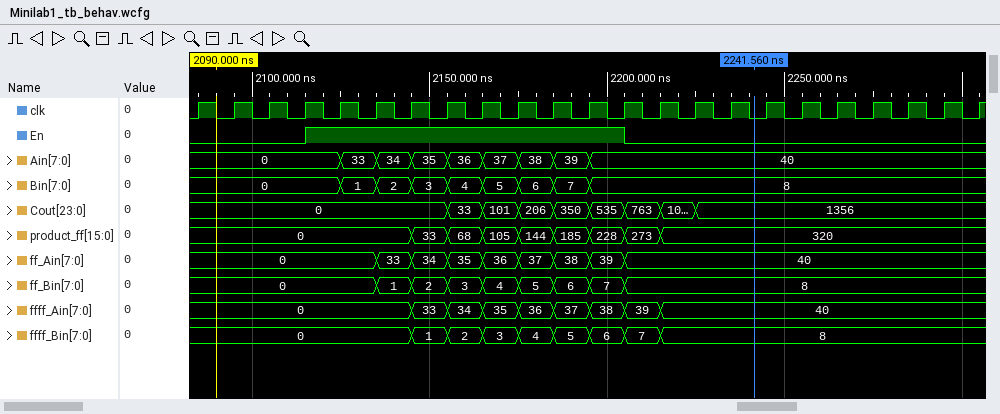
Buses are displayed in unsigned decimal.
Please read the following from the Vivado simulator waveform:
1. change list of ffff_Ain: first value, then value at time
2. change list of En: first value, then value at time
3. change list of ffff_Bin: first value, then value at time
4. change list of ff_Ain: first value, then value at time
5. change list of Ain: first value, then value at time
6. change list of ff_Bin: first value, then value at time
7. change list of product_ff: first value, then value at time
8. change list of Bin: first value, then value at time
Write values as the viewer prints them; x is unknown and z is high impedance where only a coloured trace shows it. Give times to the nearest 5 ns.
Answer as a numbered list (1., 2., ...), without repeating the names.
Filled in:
1. 0, 33 at 2145 ns, 34 at 2155 ns, 35 at 2165 ns, 36 at 2175 ns, 37 at 2185 ns, 38 at 2195 ns, 39 at 2205 ns, 40 at 2215 ns
2. 0, 1 at 2115 ns, 0 at 2205 ns
3. 0, 1 at 2145 ns, 2 at 2155 ns, 3 at 2165 ns, 4 at 2175 ns, 5 at 2185 ns, 6 at 2195 ns, 7 at 2205 ns, 8 at 2215 ns
4. 0, 33 at 2135 ns, 34 at 2145 ns, 35 at 2155 ns, 36 at 2165 ns, 37 at 2175 ns, 38 at 2185 ns, 39 at 2195 ns, 40 at 2205 ns
5. 0, 33 at 2125 ns, 34 at 2135 ns, 35 at 2145 ns, 36 at 2155 ns, 37 at 2165 ns, 38 at 2175 ns, 39 at 2185 ns, 40 at 2195 ns
6. 0, 1 at 2135 ns, 2 at 2145 ns, 3 at 2155 ns, 4 at 2165 ns, 5 at 2175 ns, 6 at 2185 ns, 7 at 2195 ns, 8 at 2205 ns
7. 0, 33 at 2145 ns, 68 at 2155 ns, 105 at 2165 ns, 144 at 2175 ns, 185 at 2185 ns, 228 at 2195 ns, 273 at 2205 ns, 320 at 2215 ns
8. 0, 1 at 2125 ns, 2 at 2135 ns, 3 at 2145 ns, 4 at 2155 ns, 5 at 2165 ns, 6 at 2175 ns, 7 at 2185 ns, 8 at 2195 ns
